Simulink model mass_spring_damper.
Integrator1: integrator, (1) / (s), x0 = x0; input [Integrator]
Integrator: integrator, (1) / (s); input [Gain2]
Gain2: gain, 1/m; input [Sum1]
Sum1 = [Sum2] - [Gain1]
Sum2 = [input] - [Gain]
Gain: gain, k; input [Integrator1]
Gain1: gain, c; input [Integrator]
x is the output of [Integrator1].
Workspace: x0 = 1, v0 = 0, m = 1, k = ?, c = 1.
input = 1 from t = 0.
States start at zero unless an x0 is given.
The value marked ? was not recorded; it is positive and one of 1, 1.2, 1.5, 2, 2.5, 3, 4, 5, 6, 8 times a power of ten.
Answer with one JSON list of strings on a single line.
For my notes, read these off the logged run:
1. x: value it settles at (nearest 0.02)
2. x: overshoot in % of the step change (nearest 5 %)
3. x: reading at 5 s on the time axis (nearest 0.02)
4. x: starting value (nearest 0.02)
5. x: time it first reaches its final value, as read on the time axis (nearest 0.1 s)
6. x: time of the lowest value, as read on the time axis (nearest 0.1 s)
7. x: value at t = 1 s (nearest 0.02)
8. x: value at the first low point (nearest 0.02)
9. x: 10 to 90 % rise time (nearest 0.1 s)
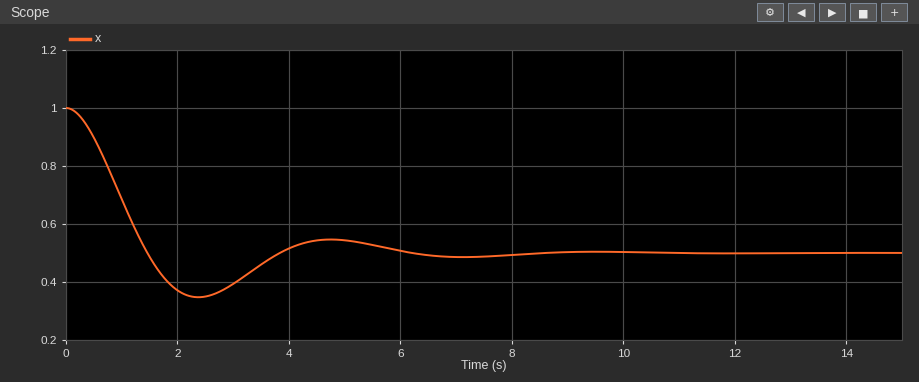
["0.50", "30 %", "0.54", "1.00", "1.5 s", "2.4 s", "0.68", "0.34", "1.0 s"]
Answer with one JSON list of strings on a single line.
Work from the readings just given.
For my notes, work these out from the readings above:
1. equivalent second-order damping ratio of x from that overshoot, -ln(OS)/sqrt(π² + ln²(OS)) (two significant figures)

["0.36"]
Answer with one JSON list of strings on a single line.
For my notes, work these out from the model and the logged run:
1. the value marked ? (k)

["2"]
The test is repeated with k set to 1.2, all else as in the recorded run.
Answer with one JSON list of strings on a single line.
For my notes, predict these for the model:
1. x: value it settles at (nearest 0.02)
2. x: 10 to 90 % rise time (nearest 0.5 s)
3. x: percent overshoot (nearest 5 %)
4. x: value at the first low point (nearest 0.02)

["0.84", "1.5 s", "20 %", "0.80"]
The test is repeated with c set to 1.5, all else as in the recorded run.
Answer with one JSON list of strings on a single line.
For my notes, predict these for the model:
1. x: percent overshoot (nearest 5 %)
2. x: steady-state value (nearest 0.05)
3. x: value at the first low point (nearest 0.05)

["15 %", "0.50", "0.45"]
